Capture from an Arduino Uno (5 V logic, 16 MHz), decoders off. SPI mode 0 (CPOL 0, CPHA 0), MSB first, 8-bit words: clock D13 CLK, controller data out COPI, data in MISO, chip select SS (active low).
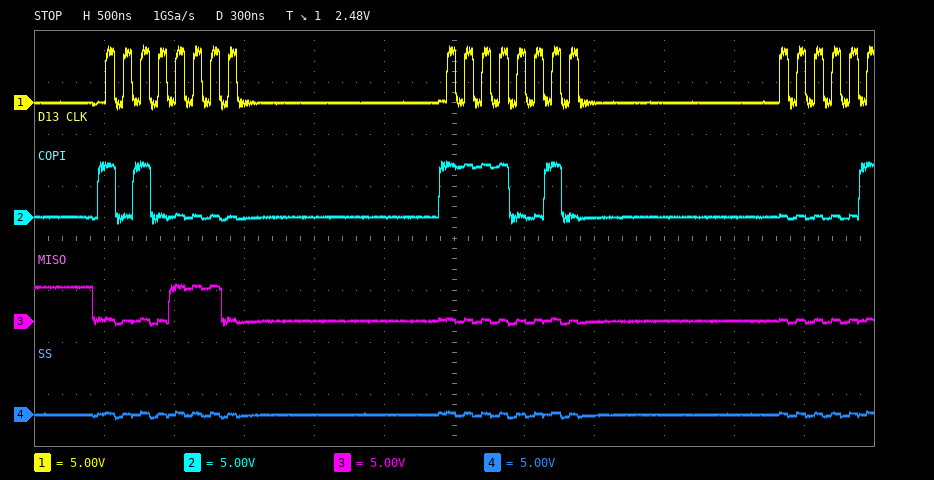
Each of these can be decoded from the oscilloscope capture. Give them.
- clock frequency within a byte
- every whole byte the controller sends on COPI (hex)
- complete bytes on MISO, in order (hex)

8 MHz
A0 F2
0E 00
